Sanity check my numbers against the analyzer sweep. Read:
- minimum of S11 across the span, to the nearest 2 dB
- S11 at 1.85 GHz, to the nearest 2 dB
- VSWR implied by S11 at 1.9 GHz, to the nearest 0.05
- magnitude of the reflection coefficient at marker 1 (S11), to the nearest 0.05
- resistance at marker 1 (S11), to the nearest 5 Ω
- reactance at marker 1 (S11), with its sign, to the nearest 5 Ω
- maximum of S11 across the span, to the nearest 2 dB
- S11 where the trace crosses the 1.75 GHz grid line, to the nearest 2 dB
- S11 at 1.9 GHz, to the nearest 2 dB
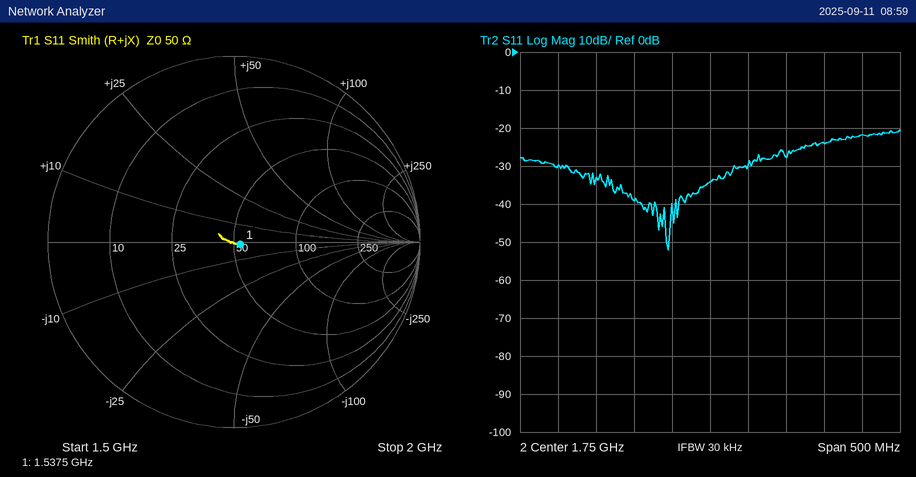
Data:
-52 dB
-28 dB
1.15
0.05
55 Ω
0 Ω
-20 dB
-34 dB
-24 dB
